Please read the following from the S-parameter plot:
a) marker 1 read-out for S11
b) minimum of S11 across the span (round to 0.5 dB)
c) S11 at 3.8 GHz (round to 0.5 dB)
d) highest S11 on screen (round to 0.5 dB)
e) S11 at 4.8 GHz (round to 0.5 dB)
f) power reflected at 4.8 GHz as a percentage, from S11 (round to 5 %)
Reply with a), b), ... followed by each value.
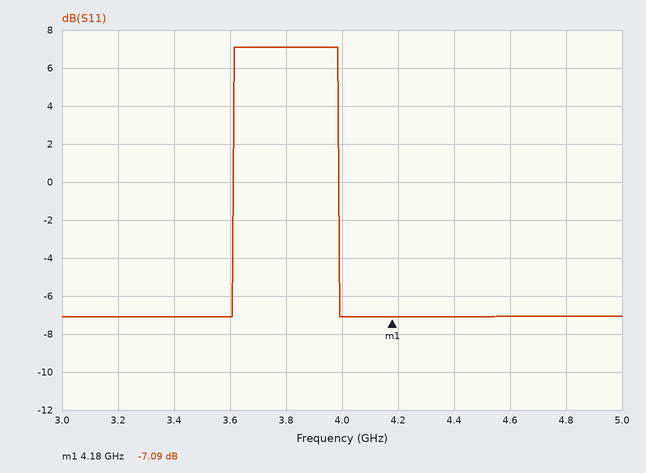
a) -7.09 dB
b) -7.0 dB
c) 7.0 dB
d) 7.0 dB
e) -7.0 dB
f) 20 %
